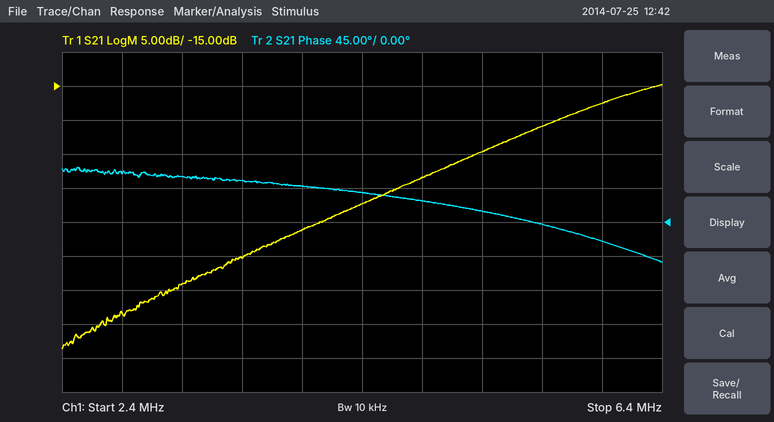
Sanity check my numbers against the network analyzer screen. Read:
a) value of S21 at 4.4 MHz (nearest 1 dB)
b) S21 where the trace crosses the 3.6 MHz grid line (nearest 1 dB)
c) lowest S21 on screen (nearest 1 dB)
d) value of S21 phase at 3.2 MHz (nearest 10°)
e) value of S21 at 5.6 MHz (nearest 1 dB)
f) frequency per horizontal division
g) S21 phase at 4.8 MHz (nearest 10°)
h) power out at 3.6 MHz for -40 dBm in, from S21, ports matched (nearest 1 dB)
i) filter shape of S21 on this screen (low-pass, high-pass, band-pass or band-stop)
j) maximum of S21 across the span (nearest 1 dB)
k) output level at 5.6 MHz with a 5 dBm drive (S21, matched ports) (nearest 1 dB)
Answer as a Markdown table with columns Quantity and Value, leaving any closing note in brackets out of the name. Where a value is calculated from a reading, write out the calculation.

| Quantity | Value |
|---|---|
| value of S21 at 4.4 MHz | -32 dB |
| S21 where the trace crosses the 3.6 MHz grid line | -40 dB |
| lowest S21 on screen | -54 dB |
| value of S21 phase at 3.2 MHz | 60° |
| value of S21 at 5.6 MHz | -21 dB |
| frequency per horizontal division | 400 kHz |
| S21 phase at 4.8 MHz | 30° |
| power out at 3.6 MHz for -40 dBm in, from S21, ports matched | -40 dBm + (-40 dB) = -80 dBm |
| filter shape of S21 on this screen | high-pass |
| maximum of S21 across the span | -15 dB |
| output level at 5.6 MHz with a 5 dBm drive (S21, matched ports) | 5 dBm + (-21 dB) = -16 dBm |
